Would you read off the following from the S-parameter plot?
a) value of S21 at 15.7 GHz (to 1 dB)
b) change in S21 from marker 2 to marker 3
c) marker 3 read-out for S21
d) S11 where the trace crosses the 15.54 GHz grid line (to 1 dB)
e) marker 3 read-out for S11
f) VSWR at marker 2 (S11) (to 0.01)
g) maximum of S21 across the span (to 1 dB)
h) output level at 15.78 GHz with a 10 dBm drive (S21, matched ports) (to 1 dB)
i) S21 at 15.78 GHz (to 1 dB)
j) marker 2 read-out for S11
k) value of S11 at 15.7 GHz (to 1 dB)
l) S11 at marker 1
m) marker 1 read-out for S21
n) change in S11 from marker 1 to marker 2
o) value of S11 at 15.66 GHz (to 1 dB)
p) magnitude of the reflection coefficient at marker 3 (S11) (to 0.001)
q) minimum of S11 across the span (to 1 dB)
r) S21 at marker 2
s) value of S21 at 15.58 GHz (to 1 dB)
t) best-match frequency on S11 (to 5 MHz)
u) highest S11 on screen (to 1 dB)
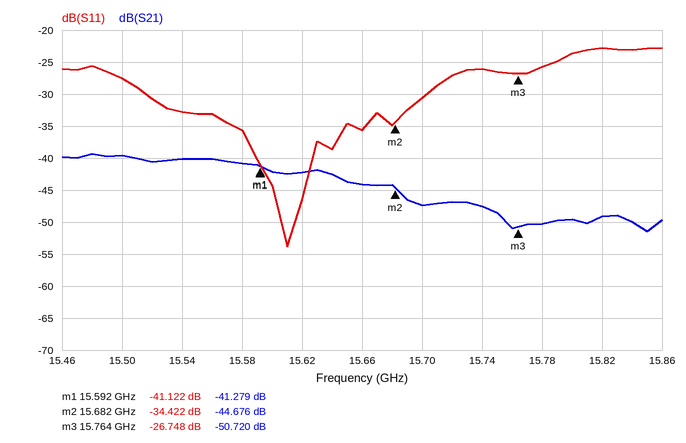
-47 dB
-6.044 dB
-50.720 dB
-33 dB
-26.748 dB
1.04
-39 dB
-40 dBm
-50 dB
-34.422 dB
-31 dB
-41.122 dB
-41.279 dB
6.700 dB
-36 dB
0.046
-54 dB
-44.676 dB
-41 dB
15.610 GHz
-23 dB
